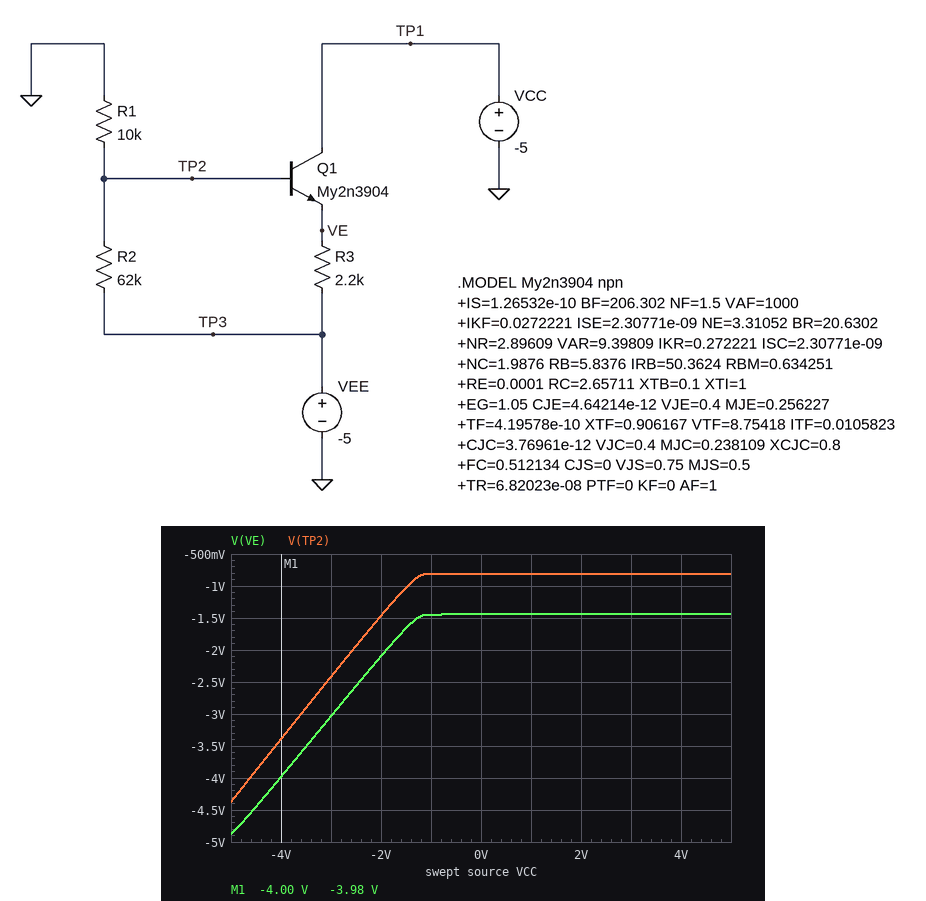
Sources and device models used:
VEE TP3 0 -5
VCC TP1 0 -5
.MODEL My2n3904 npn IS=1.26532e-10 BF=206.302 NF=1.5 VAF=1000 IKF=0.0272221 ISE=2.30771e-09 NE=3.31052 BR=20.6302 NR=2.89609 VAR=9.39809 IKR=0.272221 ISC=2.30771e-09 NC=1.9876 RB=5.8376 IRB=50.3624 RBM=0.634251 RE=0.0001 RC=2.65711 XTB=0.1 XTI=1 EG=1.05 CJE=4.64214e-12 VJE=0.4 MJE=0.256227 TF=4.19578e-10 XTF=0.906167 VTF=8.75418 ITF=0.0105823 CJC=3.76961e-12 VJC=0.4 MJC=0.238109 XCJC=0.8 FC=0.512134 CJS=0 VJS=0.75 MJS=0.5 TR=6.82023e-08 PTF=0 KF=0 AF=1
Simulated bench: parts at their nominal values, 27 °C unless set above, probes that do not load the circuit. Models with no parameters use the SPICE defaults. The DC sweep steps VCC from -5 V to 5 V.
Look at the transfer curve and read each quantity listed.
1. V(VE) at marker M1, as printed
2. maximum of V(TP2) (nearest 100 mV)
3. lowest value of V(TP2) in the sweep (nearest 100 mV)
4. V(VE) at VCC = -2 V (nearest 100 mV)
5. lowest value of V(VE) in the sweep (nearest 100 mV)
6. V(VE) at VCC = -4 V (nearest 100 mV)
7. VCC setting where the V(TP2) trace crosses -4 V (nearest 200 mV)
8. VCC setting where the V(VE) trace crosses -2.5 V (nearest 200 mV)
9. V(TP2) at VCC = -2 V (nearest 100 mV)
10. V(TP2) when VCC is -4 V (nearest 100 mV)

-3.98 V
-800 mV
-4.4 V
-2.1 V
-4.9 V
-4.0 V
-4.6 V
-2.4 V
-1.5 V
-3.4 V
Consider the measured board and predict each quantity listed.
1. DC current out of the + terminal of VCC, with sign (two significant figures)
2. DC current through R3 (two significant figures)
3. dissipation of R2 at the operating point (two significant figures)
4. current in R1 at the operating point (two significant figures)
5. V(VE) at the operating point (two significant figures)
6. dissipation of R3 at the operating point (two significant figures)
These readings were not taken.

-370 µA
54 µA
6.3 µW
440 µA
-4.9 V
6.5 µW
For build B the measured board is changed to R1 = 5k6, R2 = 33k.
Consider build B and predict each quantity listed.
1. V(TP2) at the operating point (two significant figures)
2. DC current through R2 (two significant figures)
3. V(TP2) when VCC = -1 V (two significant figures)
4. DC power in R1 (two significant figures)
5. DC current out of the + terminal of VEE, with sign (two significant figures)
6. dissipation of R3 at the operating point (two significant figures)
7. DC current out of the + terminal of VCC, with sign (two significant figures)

-4.3 V
20 µA
-790 mV
3.4 mW
-85 µA
9.2 µW
-690 µA
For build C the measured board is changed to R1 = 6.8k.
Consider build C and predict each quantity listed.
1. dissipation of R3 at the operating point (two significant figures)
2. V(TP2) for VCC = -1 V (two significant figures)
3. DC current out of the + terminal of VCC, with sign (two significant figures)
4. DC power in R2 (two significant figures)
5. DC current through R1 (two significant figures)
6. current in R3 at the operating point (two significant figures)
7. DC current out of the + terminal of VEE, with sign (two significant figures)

8.3 µW
-610 mV
-570 µA
6.8 µW
640 µA
61 µA
-72 µA
